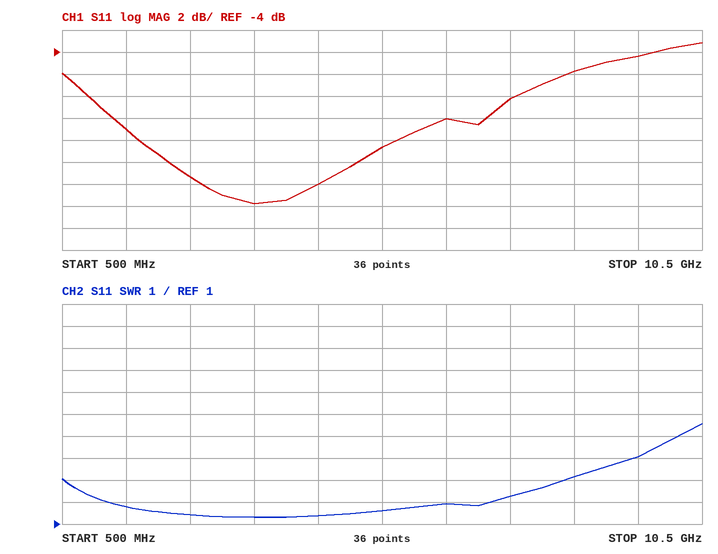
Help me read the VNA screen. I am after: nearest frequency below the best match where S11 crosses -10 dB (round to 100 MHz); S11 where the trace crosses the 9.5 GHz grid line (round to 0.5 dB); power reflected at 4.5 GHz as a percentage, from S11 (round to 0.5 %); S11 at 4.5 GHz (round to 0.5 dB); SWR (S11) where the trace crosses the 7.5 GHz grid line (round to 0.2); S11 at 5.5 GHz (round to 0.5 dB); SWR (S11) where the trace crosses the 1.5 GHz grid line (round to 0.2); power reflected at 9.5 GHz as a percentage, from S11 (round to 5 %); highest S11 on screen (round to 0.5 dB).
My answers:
1.3 GHz
-4.5 dB
2.5 %
-16.0 dB
2.2
-12.5 dB
1.8
35 %
-3.0 dB
